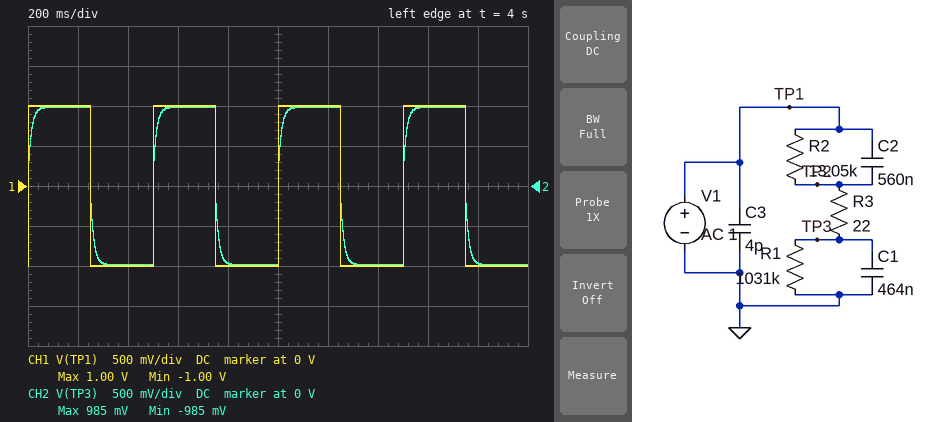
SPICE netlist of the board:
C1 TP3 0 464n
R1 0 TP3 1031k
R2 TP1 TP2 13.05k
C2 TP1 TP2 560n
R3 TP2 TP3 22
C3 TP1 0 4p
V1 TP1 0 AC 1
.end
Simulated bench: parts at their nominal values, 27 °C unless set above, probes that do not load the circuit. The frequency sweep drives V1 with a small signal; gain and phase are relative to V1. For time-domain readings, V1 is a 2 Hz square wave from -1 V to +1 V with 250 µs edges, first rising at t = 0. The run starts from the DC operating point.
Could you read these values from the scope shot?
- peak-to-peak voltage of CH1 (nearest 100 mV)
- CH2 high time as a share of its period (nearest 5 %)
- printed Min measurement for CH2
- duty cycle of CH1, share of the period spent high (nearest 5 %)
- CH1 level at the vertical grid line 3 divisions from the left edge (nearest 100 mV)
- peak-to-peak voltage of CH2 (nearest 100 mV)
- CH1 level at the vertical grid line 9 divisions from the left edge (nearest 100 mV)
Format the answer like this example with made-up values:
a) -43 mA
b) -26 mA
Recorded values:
a) 2.0 V
b) 50 %
c) -985 mV
d) 50 %
e) 1.0 V
f) 2.0 V
g) -1.0 V
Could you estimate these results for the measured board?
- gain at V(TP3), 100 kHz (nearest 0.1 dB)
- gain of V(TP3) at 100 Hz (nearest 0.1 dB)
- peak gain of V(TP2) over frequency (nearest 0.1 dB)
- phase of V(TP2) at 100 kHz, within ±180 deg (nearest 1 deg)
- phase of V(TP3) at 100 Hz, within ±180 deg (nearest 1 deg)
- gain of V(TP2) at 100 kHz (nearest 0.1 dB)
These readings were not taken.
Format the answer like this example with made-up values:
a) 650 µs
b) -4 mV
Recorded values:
a) -16.5 dB
b) -5.1 dB
c) 0 dB
d) 7 deg
e) -6 deg
f) -0.2 dB
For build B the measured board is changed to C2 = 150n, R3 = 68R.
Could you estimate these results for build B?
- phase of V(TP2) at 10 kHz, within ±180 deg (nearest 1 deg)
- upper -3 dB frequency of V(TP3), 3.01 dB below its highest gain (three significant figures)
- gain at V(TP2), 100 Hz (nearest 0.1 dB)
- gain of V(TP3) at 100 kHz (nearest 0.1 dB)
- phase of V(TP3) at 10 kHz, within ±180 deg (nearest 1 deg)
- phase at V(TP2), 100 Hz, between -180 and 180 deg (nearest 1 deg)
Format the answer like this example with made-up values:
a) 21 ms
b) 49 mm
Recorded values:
a) 37 deg
b) 21.4 Hz
c) -10.2 dB
d) -26.1 dB
e) -26 deg
f) -27 deg
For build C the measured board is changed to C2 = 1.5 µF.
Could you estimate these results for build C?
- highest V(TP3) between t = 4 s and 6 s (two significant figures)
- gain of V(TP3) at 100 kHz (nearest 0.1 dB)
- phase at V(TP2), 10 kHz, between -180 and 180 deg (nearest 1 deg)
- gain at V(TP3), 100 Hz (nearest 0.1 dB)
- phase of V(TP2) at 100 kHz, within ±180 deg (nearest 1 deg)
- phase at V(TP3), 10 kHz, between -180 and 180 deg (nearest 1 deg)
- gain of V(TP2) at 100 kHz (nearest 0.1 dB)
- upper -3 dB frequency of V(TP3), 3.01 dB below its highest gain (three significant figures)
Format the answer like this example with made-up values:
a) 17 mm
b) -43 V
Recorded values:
a) 990 mV
b) -16.3 dB
c) 7 deg
d) -2.3 dB
e) 3 deg
f) -26 deg
g) -0.1 dB
h) 9.04 kHz
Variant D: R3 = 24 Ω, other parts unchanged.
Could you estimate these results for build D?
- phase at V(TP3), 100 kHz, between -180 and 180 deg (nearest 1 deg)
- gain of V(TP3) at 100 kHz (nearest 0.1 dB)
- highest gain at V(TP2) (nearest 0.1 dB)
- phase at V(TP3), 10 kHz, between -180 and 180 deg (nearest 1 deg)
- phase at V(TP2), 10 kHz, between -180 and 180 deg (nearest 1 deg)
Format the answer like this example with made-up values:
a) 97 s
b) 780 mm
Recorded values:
a) -75 deg
b) -17.2 dB
c) 0 dB
d) -21 deg
e) 14 deg
